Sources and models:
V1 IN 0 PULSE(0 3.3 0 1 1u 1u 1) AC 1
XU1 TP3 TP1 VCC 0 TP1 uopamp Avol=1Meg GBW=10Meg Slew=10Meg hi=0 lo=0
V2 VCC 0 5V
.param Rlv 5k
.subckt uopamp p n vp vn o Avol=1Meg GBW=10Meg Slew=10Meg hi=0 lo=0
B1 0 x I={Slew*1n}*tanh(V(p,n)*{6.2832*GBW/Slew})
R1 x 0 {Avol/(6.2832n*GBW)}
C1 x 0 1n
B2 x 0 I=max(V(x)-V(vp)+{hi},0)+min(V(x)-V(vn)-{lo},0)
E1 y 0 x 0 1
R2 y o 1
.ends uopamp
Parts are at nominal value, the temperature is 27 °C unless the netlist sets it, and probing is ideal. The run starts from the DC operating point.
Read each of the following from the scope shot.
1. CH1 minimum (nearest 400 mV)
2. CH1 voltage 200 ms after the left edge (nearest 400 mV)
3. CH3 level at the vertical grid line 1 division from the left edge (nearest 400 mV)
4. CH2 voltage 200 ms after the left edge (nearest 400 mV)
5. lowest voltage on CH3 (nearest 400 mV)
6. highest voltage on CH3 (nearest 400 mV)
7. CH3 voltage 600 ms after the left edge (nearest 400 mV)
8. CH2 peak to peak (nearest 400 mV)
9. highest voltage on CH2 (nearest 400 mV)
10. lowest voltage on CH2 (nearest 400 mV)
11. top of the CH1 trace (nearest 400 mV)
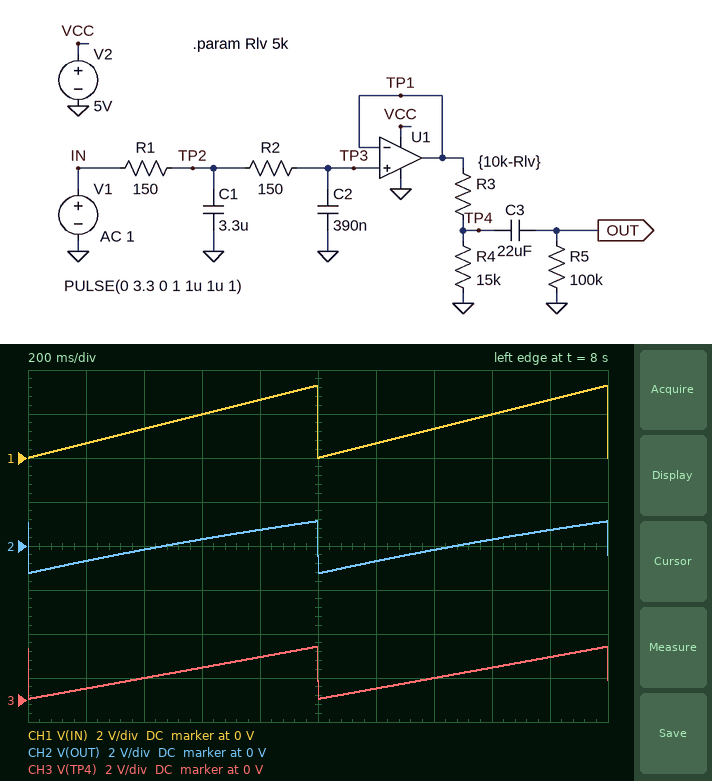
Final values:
0 V
800 mV
400 mV
-800 mV
0 V
2.4 V
1.6 V
2.4 V
1.2 V
-1.2 V
3.2 V
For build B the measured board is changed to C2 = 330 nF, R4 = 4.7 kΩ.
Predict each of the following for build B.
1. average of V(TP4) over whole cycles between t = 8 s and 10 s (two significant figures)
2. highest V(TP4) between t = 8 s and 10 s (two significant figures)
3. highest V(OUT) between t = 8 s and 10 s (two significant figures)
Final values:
800 mV
1.6 V
740 mV
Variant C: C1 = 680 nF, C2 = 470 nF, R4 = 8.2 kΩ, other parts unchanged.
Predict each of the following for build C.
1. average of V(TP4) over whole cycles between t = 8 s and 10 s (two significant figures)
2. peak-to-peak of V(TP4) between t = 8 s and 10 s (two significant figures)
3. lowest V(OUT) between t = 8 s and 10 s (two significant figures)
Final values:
1.0 V
2.0 V
-1.0 V
